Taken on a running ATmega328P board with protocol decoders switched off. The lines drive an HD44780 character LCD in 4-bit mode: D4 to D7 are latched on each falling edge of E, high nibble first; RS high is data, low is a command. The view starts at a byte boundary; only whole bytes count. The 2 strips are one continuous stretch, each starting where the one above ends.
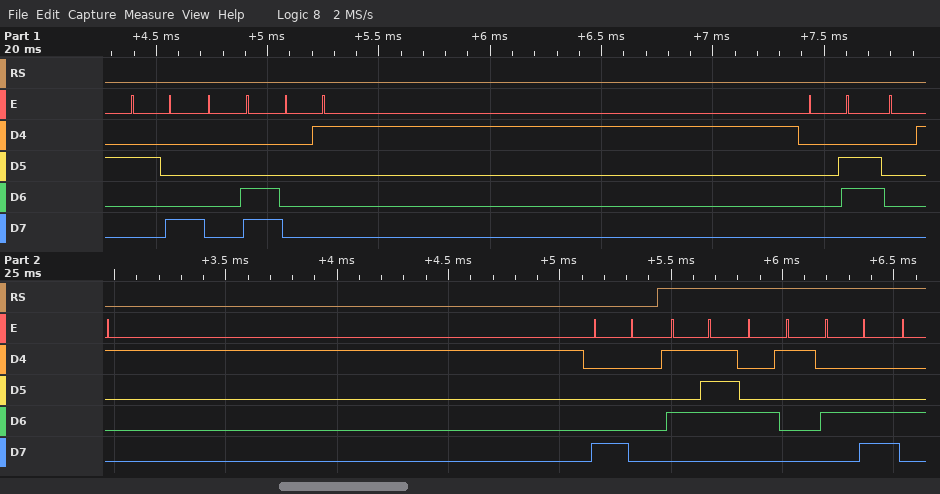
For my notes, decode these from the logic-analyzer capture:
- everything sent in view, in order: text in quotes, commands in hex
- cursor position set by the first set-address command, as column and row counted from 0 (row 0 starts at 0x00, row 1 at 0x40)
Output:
0x28 0x0C 0x01 0x06 0x01 0x80 "WAL"
column 0, row 0
